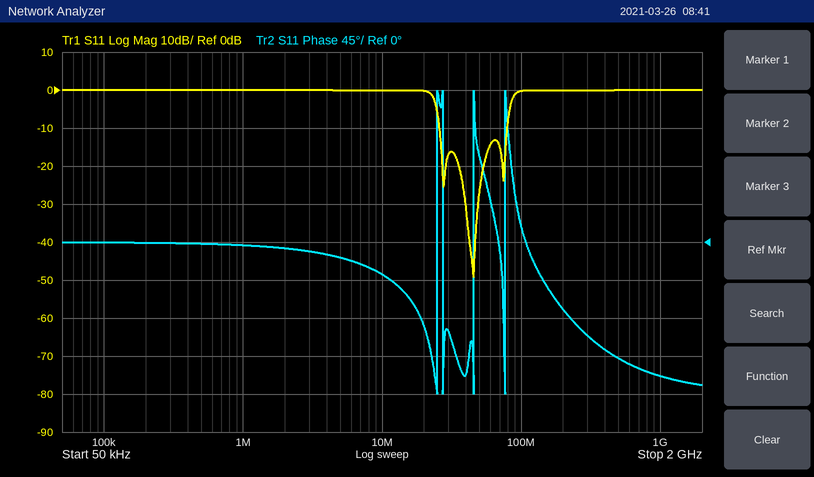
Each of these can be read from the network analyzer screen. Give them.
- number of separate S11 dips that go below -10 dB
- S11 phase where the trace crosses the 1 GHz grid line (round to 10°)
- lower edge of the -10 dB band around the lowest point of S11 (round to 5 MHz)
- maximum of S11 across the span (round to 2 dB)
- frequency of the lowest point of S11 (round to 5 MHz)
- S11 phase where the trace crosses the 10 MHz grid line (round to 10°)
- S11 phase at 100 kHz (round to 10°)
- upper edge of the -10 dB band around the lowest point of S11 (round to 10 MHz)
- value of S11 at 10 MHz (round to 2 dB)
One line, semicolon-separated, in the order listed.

3; -160°; 25 MHz; 0 dB; 45 MHz; -40°; 0°; 80 MHz; 0 dB
